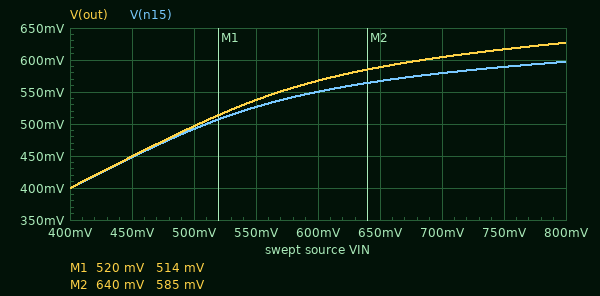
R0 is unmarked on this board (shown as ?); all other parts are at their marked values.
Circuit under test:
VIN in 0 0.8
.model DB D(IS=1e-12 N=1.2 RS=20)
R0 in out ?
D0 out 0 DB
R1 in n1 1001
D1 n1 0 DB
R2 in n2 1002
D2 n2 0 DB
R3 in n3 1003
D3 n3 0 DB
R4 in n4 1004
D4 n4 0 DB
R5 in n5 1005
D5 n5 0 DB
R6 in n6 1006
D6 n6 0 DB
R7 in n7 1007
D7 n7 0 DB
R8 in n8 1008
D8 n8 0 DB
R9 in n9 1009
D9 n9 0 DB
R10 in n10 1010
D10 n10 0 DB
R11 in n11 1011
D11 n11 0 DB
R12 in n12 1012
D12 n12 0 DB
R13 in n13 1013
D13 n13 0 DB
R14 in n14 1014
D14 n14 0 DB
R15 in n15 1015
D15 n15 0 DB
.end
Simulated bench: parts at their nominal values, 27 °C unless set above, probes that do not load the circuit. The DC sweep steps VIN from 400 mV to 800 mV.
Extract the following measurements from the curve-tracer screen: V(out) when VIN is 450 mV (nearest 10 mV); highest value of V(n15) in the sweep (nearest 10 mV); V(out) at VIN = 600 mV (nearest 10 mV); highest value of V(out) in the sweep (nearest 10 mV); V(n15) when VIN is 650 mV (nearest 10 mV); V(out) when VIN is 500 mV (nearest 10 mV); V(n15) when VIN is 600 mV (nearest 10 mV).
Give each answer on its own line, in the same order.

450 mV
600 mV
570 mV
630 mV
570 mV
500 mV
550 mV
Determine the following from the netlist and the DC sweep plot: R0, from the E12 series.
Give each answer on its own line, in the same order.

390 Ω
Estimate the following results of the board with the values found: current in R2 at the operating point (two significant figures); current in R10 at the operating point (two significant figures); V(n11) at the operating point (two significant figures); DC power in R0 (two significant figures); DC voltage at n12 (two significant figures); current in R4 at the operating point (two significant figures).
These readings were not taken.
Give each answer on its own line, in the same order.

200 µA
200 µA
600 mV
77 µW
600 mV
200 µA
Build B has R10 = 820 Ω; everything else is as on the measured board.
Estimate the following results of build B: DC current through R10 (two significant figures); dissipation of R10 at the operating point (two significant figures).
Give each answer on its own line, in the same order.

240 µA
47 µW
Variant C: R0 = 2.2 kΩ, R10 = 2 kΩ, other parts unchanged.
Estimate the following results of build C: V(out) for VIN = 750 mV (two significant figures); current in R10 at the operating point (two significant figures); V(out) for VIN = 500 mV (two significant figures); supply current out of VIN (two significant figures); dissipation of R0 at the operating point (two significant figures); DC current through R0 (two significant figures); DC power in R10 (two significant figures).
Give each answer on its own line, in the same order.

570 mV
110 µA
490 mV
3.0 mA
23 µW
100 µA
25 µW
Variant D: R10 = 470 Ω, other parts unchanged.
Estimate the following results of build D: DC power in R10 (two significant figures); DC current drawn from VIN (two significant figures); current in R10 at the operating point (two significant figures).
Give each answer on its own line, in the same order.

68 µW
3.6 mA
380 µA
